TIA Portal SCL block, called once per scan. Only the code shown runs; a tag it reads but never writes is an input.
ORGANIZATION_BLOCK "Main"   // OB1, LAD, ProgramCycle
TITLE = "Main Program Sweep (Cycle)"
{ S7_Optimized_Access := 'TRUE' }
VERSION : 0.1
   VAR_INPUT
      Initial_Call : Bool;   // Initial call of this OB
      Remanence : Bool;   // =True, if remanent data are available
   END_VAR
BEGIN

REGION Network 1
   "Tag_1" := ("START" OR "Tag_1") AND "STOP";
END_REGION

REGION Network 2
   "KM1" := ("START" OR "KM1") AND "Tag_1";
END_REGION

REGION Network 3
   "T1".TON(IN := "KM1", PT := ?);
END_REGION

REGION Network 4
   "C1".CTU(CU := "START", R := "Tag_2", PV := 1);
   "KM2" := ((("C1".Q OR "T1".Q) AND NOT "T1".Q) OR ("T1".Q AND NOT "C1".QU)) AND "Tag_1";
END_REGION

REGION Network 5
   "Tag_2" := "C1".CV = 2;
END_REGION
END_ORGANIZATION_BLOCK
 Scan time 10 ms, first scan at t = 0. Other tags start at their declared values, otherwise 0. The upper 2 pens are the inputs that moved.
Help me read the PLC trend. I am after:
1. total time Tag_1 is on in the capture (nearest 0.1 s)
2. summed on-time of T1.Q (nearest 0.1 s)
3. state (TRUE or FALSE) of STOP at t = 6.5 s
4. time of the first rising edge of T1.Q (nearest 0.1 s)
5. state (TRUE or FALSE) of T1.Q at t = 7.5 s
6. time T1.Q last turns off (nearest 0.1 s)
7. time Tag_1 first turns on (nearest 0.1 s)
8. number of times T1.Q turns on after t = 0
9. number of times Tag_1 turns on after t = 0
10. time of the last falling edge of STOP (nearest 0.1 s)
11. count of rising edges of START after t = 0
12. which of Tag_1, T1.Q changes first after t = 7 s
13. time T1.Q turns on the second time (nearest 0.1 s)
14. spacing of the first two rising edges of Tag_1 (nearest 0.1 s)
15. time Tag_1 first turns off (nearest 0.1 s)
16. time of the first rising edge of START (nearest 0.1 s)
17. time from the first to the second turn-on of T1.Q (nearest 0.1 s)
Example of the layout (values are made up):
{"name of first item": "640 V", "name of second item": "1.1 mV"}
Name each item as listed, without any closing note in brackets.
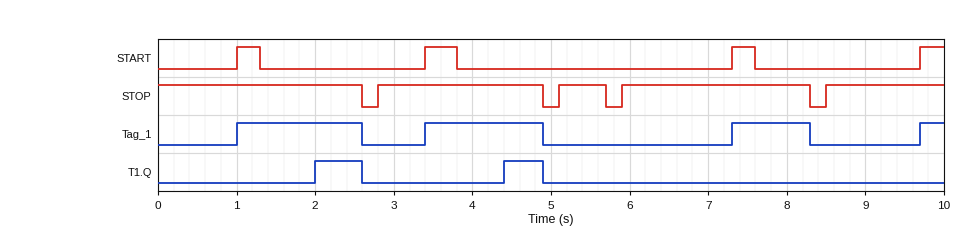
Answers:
{"total time Tag_1 is on in the capture": "4.4 s", "summed on-time of T1.Q": "1.1 s", "state (TRUE or FALSE) of STOP at t = 6.5 s": "TRUE", "time of the first rising edge of T1.Q": "2.0 s", "state (TRUE or FALSE) of T1.Q at t = 7.5 s": "FALSE", "time T1.Q last turns off": "4.9 s", "time Tag_1 first turns on": "1.0 s", "number of times T1.Q turns on after t = 0": "2", "number of times Tag_1 turns on after t = 0": "4", "time of the last falling edge of STOP": "8.3 s", "count of rising edges of START after t = 0": "4", "which of Tag_1, T1.Q changes first after t = 7 s": "Tag_1", "time T1.Q turns on the second time": "4.4 s", "spacing of the first two rising edges of Tag_1": "2.4 s", "time Tag_1 first turns off": "2.6 s", "time of the first rising edge of START": "1.0 s", "time from the first to the second turn-on of T1.Q": "2.4 s"}
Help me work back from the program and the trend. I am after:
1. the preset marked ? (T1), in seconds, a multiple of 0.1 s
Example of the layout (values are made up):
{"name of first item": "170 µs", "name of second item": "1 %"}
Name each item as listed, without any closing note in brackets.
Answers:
{"the preset marked ? (T1), in seconds, a multiple of 0.1 s": "1.0 s"}
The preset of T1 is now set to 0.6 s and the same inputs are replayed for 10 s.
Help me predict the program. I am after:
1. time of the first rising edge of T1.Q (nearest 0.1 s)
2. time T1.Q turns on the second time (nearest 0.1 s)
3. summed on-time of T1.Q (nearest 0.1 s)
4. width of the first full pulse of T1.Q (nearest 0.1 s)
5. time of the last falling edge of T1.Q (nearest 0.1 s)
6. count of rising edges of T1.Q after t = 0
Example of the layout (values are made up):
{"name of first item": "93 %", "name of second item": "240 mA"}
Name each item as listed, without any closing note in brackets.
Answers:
{"time of the first rising edge of T1.Q": "1.6 s", "time T1.Q turns on the second time": "4.0 s", "summed on-time of T1.Q": "2.3 s", "width of the first full pulse of T1.Q": "1.0 s", "time of the last falling edge of T1.Q": "8.3 s", "count of rising edges of T1.Q after t = 0": "3"}
